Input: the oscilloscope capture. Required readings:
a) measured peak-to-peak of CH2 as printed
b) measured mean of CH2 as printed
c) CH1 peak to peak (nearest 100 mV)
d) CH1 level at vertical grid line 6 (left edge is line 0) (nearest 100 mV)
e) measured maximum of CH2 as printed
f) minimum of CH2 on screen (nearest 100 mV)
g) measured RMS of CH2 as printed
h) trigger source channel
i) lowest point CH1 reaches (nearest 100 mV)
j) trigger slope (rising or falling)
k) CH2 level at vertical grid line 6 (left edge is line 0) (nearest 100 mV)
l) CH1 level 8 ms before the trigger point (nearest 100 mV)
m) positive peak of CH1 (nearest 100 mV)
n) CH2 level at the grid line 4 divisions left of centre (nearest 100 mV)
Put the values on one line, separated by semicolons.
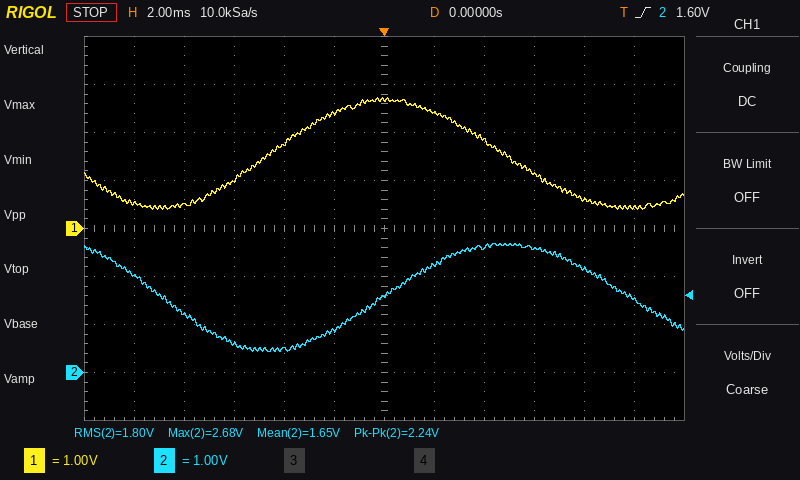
2.24 V; 1.65 V; 2.3 V; 2.7 V; 2.68 V; 400 mV; 1.80 V; CH2; 400 mV; rising; 1.6 V; 500 mV; 2.7 V; 1.2 V
